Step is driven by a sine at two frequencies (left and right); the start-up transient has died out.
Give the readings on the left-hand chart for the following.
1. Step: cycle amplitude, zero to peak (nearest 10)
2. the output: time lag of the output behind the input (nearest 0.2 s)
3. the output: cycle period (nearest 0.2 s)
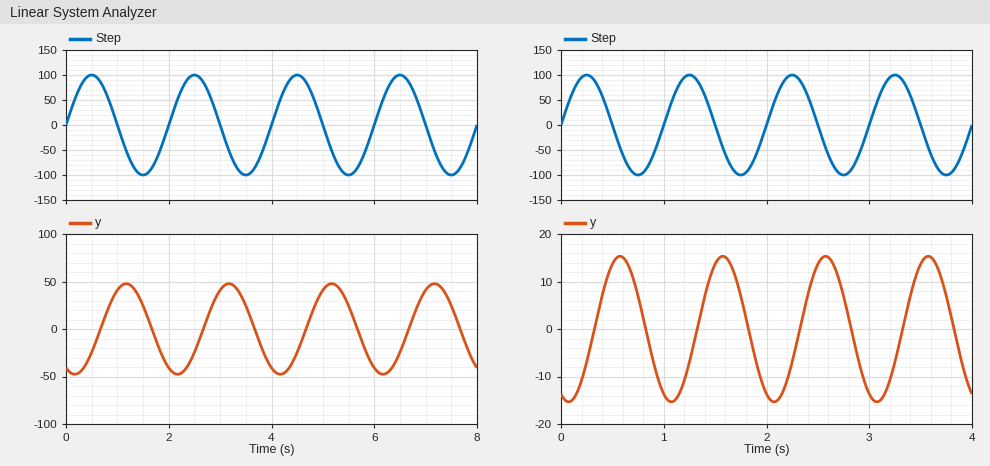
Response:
100
0.6 s
2.0 s
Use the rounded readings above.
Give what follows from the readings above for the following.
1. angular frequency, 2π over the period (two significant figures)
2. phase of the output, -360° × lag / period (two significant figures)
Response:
3.1 rad/s
-110°
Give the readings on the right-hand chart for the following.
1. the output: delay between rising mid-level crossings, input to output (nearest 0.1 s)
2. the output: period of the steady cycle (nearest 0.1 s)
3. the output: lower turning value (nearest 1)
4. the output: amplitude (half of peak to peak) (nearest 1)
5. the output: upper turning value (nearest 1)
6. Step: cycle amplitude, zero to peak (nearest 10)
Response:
0.3 s
1.0 s
-15
15
15
100
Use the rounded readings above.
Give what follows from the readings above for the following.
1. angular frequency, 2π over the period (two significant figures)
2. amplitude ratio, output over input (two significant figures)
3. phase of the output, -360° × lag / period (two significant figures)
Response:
6.3 rad/s
0.15
-110°
